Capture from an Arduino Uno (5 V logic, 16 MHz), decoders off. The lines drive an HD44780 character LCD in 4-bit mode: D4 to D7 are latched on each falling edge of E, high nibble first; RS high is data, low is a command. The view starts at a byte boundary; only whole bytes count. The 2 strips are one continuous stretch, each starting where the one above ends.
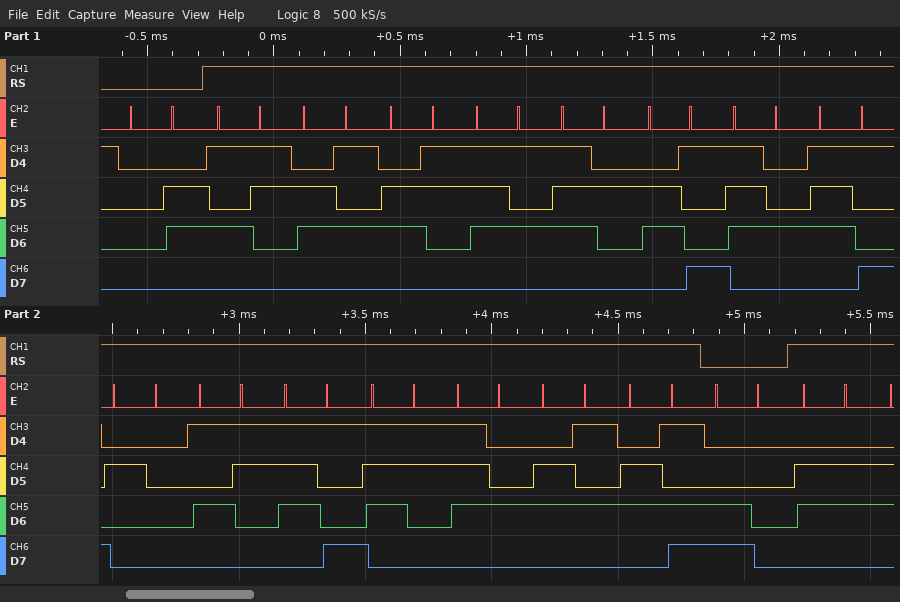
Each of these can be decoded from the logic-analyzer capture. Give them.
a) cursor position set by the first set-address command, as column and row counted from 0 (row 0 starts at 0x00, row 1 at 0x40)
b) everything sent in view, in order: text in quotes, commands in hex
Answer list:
column 0, row 1
0x06 "Security System" 0xC0 "f"
